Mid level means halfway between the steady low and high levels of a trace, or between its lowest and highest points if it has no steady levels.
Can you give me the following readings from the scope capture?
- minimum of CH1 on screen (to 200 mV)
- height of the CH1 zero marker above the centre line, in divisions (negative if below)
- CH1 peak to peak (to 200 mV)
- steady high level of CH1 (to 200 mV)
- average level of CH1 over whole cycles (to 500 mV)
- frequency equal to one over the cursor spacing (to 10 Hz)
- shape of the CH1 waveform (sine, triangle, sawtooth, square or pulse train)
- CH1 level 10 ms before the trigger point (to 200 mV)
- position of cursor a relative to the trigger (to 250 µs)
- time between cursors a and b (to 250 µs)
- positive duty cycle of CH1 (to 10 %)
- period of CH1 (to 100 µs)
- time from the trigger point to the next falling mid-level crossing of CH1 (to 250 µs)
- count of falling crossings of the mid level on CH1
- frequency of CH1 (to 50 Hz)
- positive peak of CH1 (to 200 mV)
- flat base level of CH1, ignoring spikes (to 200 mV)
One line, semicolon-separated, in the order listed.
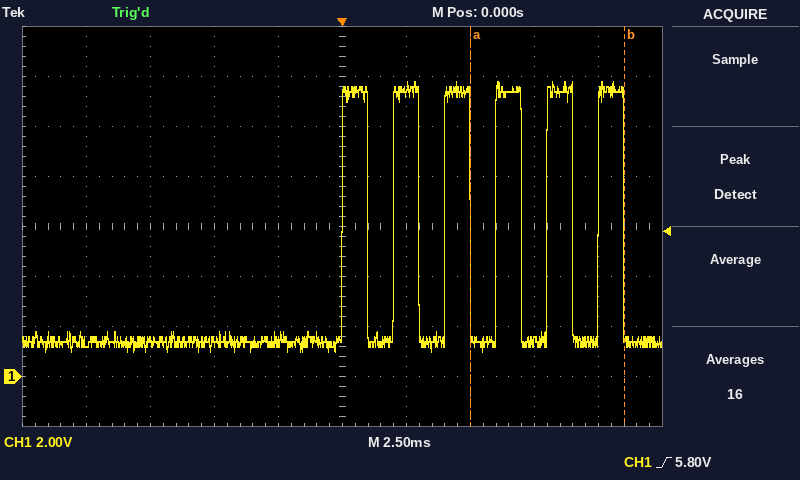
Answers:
1.0 V; -3.0 div; 10.8 V; 11.4 V; 6.5 V; 170 Hz; square; 1.4 V; +5.00 ms; 6.00 ms; 50 %; 2.0 ms; 1.00 ms; 6; 500 Hz; 11.8 V; 1.4 V
